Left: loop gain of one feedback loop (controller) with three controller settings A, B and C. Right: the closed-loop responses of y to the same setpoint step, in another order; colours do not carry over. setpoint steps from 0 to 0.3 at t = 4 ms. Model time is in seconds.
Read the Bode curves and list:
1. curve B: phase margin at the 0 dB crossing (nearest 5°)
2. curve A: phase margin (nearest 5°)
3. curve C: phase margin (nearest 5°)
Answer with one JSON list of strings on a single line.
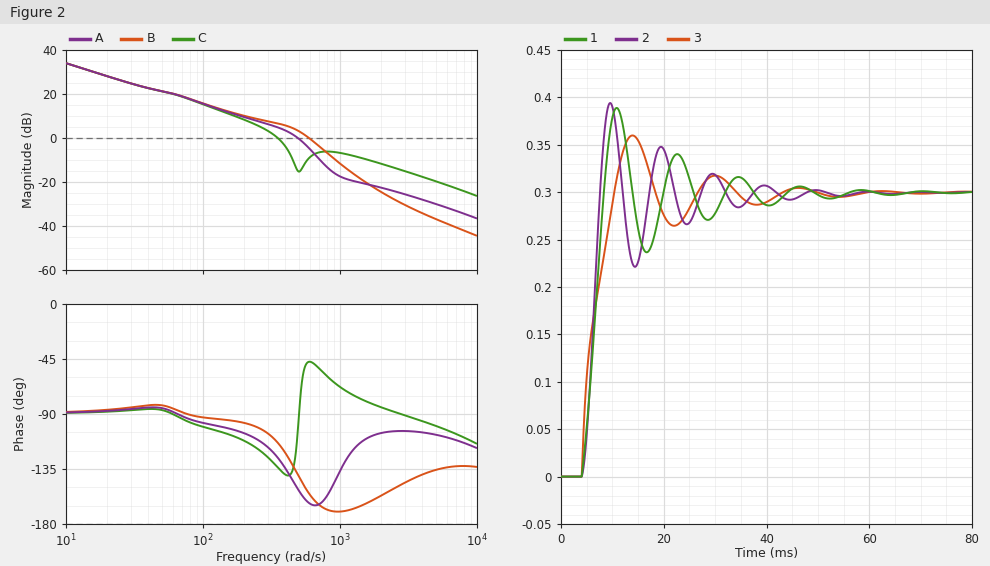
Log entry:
["25°", "30°", "45°"]
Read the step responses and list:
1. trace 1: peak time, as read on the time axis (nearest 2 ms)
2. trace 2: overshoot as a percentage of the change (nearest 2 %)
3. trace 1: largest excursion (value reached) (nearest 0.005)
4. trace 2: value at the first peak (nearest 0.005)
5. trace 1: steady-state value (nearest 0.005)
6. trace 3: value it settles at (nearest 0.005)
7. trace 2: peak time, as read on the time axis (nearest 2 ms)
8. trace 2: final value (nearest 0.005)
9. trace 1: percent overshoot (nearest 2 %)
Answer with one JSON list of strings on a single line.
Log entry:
["10 ms", "32 %", "0.390", "0.395", "0.300", "0.300", "10 ms", "0.300", "30 %"]
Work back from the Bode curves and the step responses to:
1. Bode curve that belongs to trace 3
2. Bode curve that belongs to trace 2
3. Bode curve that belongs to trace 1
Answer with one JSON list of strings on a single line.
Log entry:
["C", "B", "A"]
